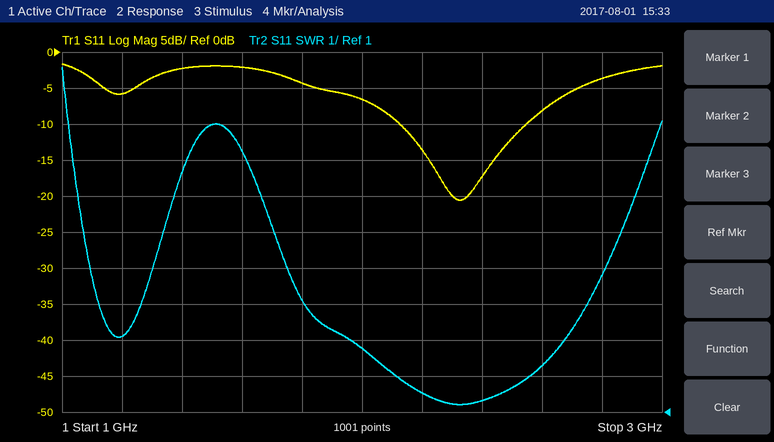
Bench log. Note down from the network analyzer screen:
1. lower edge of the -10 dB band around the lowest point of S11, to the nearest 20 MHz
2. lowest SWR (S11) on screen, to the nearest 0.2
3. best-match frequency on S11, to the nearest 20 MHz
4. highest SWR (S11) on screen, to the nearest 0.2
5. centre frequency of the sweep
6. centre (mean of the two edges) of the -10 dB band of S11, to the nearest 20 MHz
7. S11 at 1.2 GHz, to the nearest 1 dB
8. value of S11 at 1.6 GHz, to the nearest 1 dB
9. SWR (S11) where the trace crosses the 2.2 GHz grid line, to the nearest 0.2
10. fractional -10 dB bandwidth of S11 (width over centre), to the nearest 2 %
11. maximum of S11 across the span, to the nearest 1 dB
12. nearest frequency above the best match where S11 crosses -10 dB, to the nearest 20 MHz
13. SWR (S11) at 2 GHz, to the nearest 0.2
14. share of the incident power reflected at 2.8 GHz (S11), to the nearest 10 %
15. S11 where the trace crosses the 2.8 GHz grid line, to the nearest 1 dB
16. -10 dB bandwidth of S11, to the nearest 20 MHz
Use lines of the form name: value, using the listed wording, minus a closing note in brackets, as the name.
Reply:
lower edge of the -10 dB band around the lowest point of S11, to the nearest 20 MHz: 2.12 GHz
lowest SWR (S11) on screen, to the nearest 0.2: 1.2
best-match frequency on S11, to the nearest 20 MHz: 2.32 GHz
highest SWR (S11) on screen, to the nearest 0.2: 10.6
centre frequency of the sweep: 2 GHz
centre (mean of the two edges) of the -10 dB band of S11, to the nearest 20 MHz: 2.34 GHz
S11 at 1.2 GHz, to the nearest 1 dB: -6 dB
value of S11 at 1.6 GHz, to the nearest 1 dB: -2 dB
SWR (S11) where the trace crosses the 2.2 GHz grid line, to the nearest 0.2: 1.6
fractional -10 dB bandwidth of S11 (width over centre), to the nearest 2 %: 18 %
maximum of S11 across the span, to the nearest 1 dB: -2 dB
nearest frequency above the best match where S11 crosses -10 dB, to the nearest 20 MHz: 2.54 GHz
SWR (S11) at 2 GHz, to the nearest 0.2: 2.8
share of the incident power reflected at 2.8 GHz (S11), to the nearest 10 %: 40 %
S11 where the trace crosses the 2.8 GHz grid line, to the nearest 1 dB: -4 dB
-10 dB bandwidth of S11, to the nearest 20 MHz: 420 MHz
